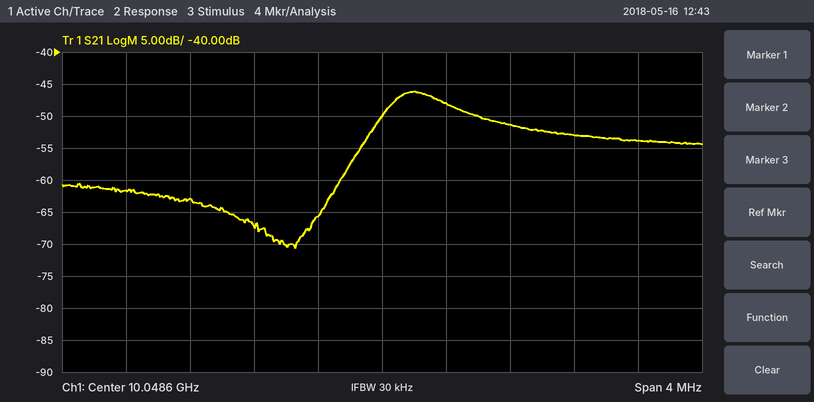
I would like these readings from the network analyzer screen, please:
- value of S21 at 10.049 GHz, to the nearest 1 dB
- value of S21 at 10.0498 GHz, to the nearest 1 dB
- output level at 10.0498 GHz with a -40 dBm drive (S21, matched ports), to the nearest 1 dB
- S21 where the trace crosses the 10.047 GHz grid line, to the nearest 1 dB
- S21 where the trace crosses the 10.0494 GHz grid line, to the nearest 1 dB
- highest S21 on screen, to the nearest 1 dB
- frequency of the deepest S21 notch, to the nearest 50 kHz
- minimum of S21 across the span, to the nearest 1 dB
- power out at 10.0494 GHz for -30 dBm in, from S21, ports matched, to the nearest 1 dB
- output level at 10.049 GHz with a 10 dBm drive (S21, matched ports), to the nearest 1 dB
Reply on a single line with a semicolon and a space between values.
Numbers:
-48 dB; -53 dB; -93 dBm; -62 dB; -51 dB; -46 dB; 10.04805 GHz; -71 dB; -81 dBm; -38 dBm
